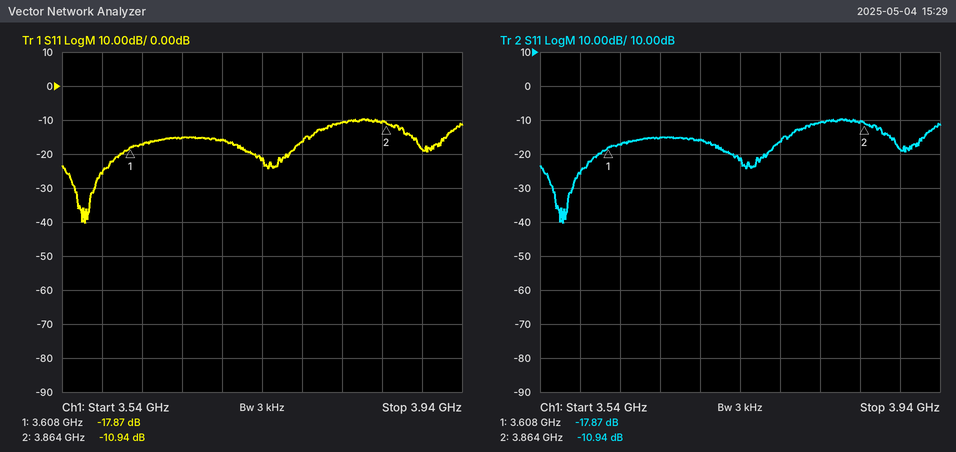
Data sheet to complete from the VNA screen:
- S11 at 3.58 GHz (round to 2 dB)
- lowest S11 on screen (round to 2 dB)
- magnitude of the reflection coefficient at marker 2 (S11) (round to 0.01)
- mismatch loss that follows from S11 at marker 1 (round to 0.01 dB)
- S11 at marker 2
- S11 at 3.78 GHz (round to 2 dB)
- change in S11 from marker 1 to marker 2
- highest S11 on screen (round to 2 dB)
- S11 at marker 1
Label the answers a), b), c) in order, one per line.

a) -26 dB
b) -40 dB
c) 0.28
d) 0.07 dB
e) -10.94 dB
f) -16 dB
g) 6.93 dB
h) -10 dB
i) -17.87 dB
